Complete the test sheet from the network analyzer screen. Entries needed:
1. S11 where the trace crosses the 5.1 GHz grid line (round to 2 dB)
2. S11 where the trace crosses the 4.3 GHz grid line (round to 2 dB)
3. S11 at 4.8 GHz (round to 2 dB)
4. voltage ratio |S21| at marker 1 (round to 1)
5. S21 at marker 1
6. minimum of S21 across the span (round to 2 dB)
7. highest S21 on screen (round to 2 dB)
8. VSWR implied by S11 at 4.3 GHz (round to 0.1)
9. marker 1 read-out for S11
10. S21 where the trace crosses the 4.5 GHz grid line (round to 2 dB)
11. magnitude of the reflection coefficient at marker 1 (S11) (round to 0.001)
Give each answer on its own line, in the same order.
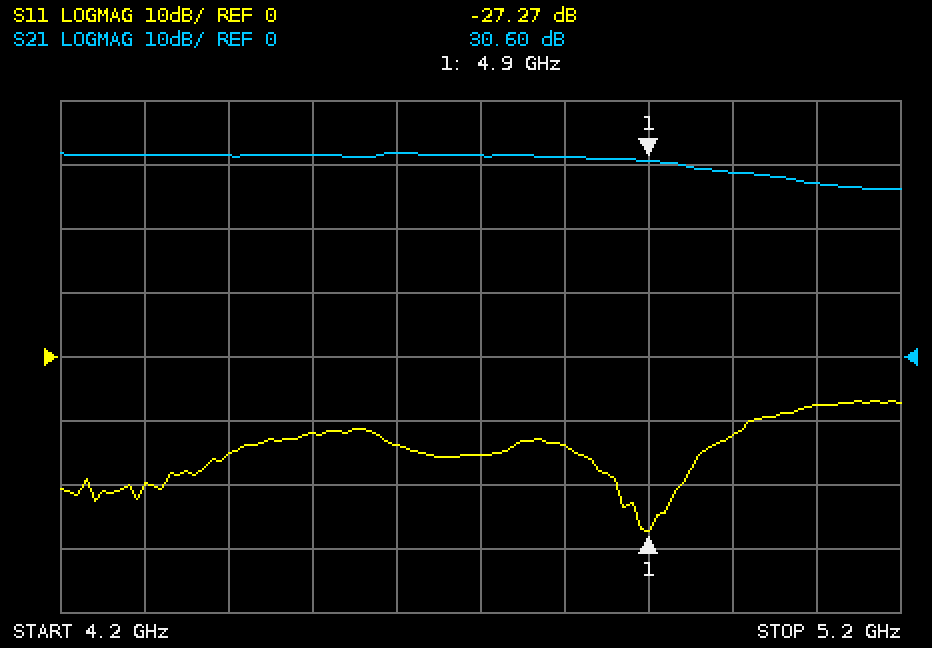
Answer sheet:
-8 dB
-20 dB
-14 dB
34
30.60 dB
26 dB
32 dB
1.2
-27.27 dB
32 dB
0.043
